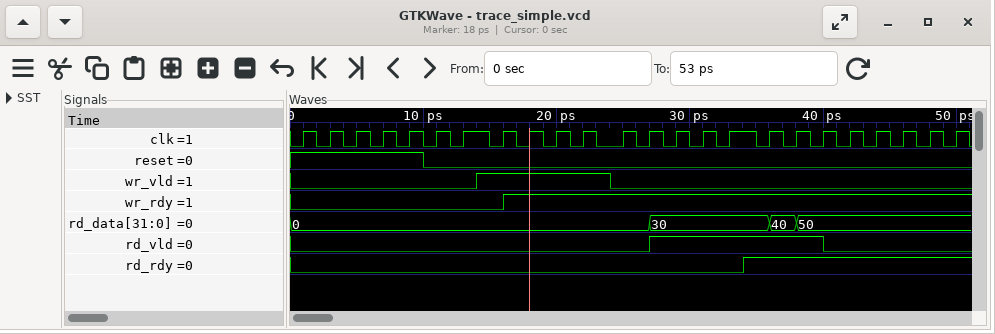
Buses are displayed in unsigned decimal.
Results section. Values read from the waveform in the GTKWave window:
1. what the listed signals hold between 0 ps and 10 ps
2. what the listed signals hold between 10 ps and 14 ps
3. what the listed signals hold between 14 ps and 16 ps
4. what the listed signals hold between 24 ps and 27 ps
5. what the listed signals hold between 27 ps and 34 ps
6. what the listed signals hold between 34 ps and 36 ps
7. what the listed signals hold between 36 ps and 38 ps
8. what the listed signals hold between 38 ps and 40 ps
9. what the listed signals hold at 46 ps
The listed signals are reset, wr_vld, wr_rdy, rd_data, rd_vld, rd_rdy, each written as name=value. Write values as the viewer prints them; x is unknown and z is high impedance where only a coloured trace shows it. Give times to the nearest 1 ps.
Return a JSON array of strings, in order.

["reset=1, wr_vld=0, wr_rdy=0, rd_data=0, rd_vld=0, rd_rdy=0", "reset=0, wr_vld=0, wr_rdy=0, rd_data=0, rd_vld=0, rd_rdy=0", "reset=0, wr_vld=1, wr_rdy=0, rd_data=0, rd_vld=0, rd_rdy=0", "reset=0, wr_vld=0, wr_rdy=1, rd_data=0, rd_vld=0, rd_rdy=0", "reset=0, wr_vld=0, wr_rdy=1, rd_data=30, rd_vld=1, rd_rdy=0", "reset=0, wr_vld=0, wr_rdy=1, rd_data=30, rd_vld=1, rd_rdy=1", "reset=0, wr_vld=0, wr_rdy=1, rd_data=40, rd_vld=1, rd_rdy=1", "reset=0, wr_vld=0, wr_rdy=1, rd_data=50, rd_vld=1, rd_rdy=1", "reset=0, wr_vld=0, wr_rdy=1, rd_data=50, rd_vld=0, rd_rdy=1"]
